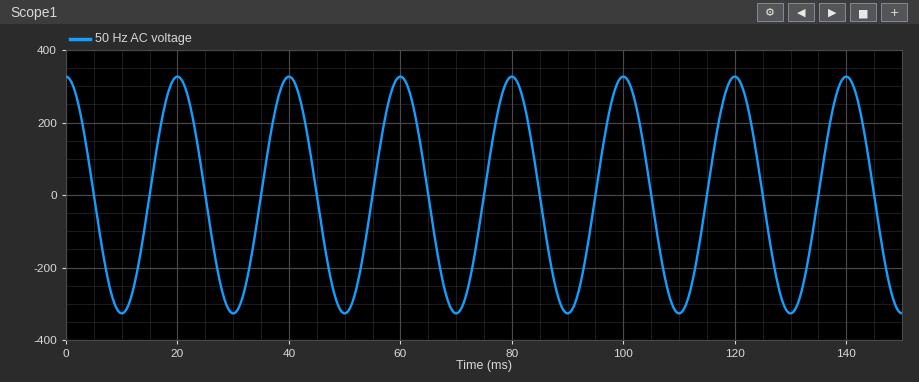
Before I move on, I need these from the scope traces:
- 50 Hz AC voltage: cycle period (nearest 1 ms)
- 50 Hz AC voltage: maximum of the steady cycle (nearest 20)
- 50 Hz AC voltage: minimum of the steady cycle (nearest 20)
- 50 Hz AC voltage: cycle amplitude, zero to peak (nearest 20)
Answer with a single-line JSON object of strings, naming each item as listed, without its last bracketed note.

{"50 Hz AC voltage: cycle period": "20 ms", "50 Hz AC voltage: maximum of the steady cycle": "320", "50 Hz AC voltage: minimum of the steady cycle": "-320", "50 Hz AC voltage: cycle amplitude, zero to peak": "320"}
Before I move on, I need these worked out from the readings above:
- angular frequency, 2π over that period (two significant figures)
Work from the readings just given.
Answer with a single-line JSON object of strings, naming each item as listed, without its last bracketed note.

{"angular frequency, 2π over that period": "0.31 rad/ms"}
